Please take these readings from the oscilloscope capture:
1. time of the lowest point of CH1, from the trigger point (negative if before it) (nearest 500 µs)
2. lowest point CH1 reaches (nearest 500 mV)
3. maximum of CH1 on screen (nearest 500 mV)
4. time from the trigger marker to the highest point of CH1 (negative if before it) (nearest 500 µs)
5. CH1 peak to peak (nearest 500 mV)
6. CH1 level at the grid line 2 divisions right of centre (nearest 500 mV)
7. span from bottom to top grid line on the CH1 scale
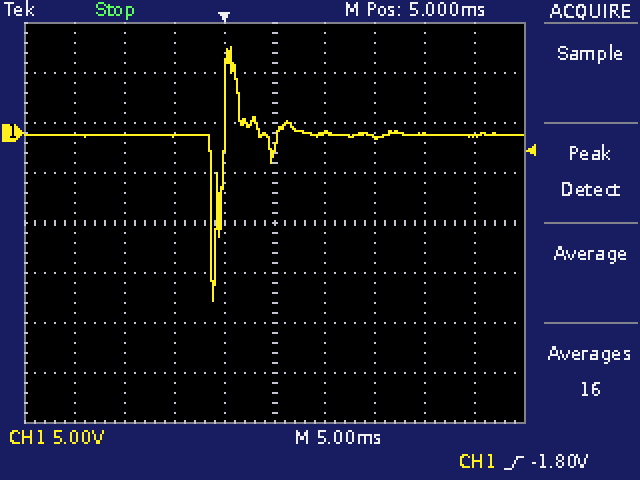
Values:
-1.0 ms
-17.0 V
8.5 V
+500 µs
25.5 V
-500 mV
40 V
